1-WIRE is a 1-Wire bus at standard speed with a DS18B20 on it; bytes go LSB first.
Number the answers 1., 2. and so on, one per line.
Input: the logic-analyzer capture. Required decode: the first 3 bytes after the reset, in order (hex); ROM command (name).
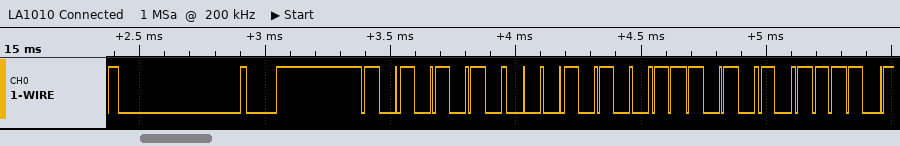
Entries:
1. 55 28 57
2. Match ROM
